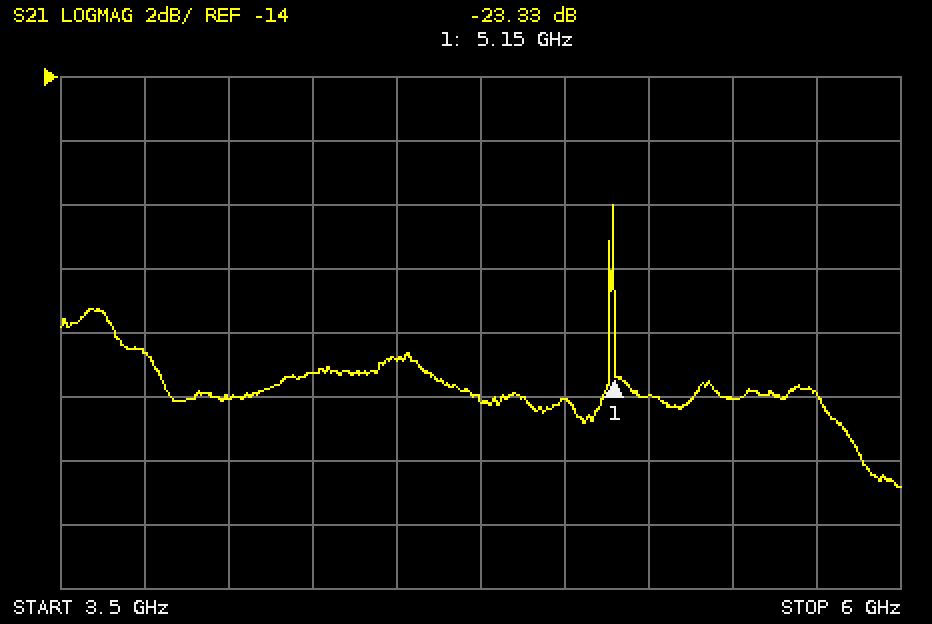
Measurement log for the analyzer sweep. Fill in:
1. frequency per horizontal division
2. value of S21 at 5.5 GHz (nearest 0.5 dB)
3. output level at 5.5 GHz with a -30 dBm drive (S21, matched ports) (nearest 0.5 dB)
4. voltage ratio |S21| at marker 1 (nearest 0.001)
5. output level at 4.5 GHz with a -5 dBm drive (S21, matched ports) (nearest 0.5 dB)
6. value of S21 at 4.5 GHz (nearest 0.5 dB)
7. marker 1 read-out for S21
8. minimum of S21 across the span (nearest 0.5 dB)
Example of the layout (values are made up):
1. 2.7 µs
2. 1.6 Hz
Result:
1. 250 MHz
2. -24.0 dB
3. -54.0 dBm
4. 0.068
5. -28.0 dBm
6. -23.0 dB
7. -23.33 dB
8. -27.0 dB
